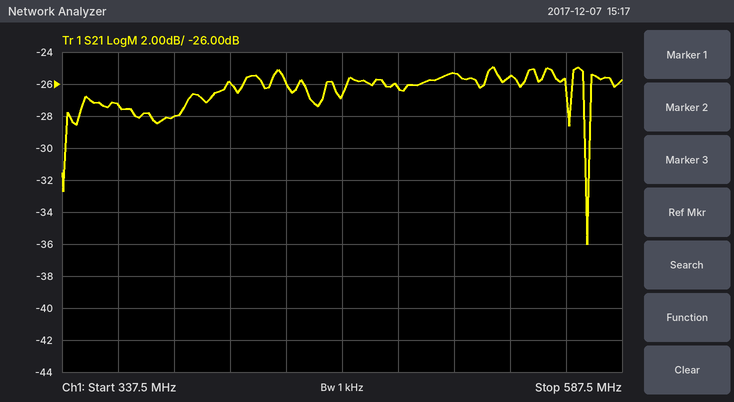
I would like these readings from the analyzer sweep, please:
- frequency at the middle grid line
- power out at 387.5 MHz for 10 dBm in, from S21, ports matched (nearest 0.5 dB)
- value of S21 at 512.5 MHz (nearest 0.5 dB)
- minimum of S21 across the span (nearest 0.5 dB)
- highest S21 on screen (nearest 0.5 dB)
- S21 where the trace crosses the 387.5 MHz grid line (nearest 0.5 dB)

462.5 MHz
-18.0 dBm
-25.5 dB
-36.0 dB
-25.0 dB
-28.0 dB
